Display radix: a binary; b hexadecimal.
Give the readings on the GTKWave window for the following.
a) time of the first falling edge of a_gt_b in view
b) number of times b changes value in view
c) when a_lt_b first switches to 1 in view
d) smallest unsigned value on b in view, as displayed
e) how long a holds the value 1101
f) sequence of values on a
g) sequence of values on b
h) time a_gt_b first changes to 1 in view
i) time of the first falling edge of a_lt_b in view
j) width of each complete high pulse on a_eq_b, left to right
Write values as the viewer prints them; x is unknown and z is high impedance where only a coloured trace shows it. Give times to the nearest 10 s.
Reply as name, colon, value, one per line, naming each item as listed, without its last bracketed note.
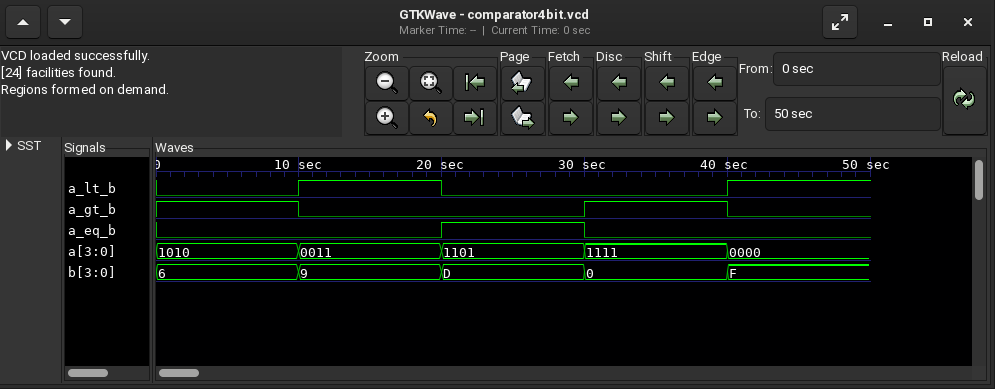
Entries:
time of the first falling edge of a_gt_b in view: 10 s
number of times b changes value in view: 4
when a_lt_b first switches to 1 in view: 10 s
smallest unsigned value on b in view, as displayed: 0
how long a holds the value 1101: 10 s
sequence of values on a: 1010, 0011, 1101, 1111, 0000
sequence of values on b: 6, 9, D, 0, F
time a_gt_b first changes to 1 in view: 30 s
time of the first falling edge of a_lt_b in view: 20 s
width of each complete high pulse on a_eq_b, left to right: 10 s
